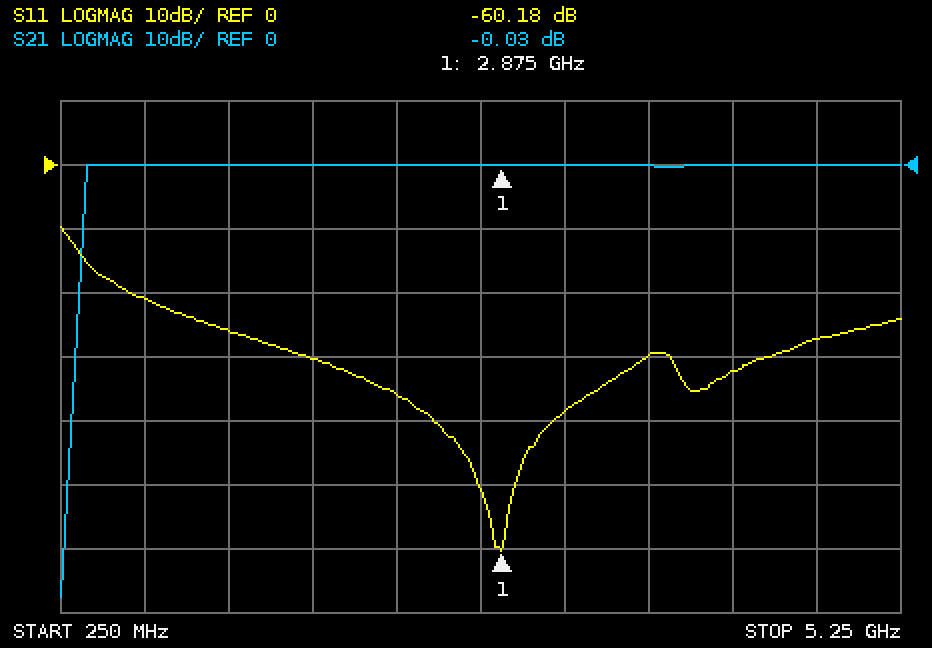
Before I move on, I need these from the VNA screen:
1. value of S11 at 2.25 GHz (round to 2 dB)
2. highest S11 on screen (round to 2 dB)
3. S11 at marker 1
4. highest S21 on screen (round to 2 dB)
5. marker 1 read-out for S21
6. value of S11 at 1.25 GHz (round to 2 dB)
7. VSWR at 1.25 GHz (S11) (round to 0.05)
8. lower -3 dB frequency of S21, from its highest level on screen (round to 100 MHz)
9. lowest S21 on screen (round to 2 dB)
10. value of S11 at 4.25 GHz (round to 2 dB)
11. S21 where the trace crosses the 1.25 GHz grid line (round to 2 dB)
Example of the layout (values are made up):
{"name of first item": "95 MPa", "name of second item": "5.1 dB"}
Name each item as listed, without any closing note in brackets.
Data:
{"value of S11 at 2.25 GHz": "-36 dB", "highest S11 on screen": "-10 dB", "S11 at marker 1": "-60.18 dB", "highest S21 on screen": "0 dB", "marker 1 read-out for S21": "-0.03 dB", "value of S11 at 1.25 GHz": "-26 dB", "VSWR at 1.25 GHz (S11)": "1.10", "lower -3 dB frequency of S21, from its highest level on screen": "400 MHz", "lowest S21 on screen": "-68 dB", "value of S11 at 4.25 GHz": "-32 dB", "S21 where the trace crosses the 1.25 GHz grid line": "0 dB"}
